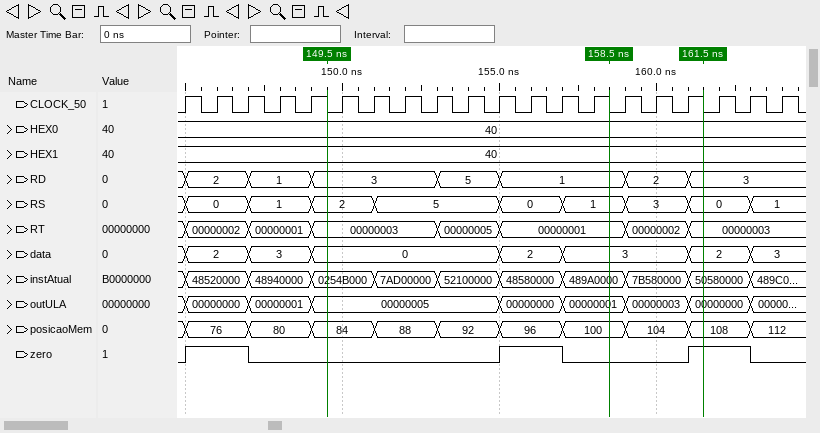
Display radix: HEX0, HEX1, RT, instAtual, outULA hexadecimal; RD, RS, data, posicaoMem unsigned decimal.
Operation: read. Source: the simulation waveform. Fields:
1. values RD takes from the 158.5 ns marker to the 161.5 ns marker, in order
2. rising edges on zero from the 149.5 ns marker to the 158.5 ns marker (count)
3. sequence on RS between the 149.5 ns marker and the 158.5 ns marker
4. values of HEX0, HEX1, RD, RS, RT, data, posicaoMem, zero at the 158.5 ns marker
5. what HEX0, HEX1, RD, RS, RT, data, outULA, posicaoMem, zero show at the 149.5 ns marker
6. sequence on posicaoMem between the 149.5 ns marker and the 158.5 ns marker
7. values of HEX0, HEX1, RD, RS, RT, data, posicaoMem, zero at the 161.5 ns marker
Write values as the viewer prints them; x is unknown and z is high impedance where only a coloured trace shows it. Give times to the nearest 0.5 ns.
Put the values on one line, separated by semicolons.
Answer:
1, 2, 3; 1; 2, 5, 0, 1; HEX0=40, HEX1=40, RD=1, RS=1, RT=00000001, data=3, posicaoMem=100, zero=0; HEX0=40, HEX1=40, RD=3, RS=2, RT=00000003, data=0, outULA=00000005, posicaoMem=84, zero=0; 84, 88, 92, 96, 100; HEX0=40, HEX1=40, RD=3, RS=0, RT=00000003, data=2, posicaoMem=108, zero=1
